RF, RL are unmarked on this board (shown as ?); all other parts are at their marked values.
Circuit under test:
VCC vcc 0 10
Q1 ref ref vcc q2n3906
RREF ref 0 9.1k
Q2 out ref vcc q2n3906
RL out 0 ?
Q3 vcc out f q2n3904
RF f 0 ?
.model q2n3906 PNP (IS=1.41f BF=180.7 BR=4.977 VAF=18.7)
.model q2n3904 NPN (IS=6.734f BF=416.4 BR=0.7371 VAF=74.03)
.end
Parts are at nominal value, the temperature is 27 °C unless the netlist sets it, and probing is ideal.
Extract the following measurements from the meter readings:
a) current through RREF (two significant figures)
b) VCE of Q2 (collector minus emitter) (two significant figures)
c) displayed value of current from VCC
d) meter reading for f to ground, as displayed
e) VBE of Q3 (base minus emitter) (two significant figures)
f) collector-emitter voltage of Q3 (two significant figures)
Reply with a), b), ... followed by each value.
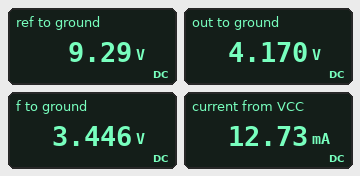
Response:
a) 1.0 mA
b) -5.8 V
c) 12.73 mA
d) 3.446 V
e) 720 mV
f) 6.6 V
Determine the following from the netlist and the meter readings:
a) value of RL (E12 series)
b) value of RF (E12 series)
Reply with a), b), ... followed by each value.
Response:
a) 3.3 kΩ
b) 330 Ω
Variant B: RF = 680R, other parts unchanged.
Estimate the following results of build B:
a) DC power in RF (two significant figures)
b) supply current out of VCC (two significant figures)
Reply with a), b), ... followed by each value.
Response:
a) 18 mW
b) 7.4 mA
